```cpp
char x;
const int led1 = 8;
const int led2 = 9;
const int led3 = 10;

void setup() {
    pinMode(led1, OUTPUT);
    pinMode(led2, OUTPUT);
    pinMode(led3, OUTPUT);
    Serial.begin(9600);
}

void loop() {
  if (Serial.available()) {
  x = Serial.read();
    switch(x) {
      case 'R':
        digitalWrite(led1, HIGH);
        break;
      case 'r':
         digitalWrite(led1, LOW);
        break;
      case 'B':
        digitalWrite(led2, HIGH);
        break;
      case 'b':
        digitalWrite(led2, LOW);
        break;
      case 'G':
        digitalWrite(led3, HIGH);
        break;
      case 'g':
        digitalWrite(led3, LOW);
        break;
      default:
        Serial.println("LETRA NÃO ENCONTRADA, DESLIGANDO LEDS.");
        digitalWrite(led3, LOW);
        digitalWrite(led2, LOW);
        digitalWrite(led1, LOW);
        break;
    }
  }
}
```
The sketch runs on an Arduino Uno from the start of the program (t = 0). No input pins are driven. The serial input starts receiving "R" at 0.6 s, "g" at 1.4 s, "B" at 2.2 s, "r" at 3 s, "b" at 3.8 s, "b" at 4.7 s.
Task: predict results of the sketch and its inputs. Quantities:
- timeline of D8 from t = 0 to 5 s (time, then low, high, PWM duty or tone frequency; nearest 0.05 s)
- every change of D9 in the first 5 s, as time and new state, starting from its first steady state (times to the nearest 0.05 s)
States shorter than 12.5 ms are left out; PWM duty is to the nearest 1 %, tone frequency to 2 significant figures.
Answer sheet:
0 s low; 0.6 s high; 3 s low
0 s low; 2.2 s high; 3.8 s low
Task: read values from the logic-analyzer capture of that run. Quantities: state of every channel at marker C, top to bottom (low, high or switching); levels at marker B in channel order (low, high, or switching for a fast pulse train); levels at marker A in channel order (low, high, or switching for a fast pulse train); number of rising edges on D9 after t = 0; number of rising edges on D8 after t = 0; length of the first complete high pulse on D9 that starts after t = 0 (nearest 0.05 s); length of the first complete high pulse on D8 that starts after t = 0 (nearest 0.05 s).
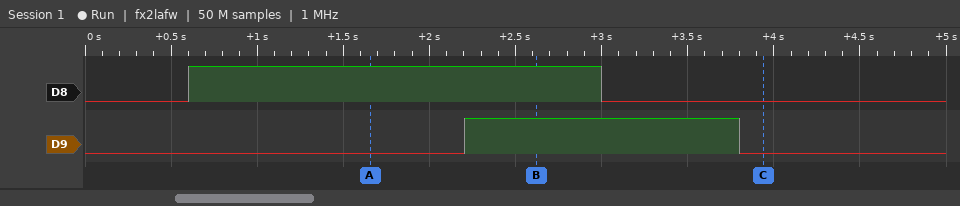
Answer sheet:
D8 low, D9 low
D8 high, D9 high
D8 high, D9 low
1
1
1.60 s
2.40 s
